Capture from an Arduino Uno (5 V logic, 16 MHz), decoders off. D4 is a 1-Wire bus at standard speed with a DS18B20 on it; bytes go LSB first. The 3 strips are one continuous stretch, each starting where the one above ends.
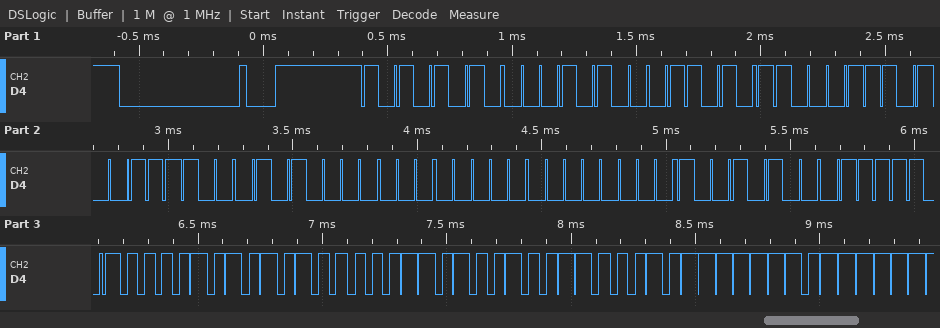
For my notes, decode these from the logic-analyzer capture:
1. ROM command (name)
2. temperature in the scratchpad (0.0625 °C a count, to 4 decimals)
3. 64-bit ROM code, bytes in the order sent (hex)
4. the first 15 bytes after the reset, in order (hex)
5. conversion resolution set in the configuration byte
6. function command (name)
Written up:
Match ROM
85.0000 °C
28 D6 B8 3C 0A 00 00 29
55 28 D6 B8 3C 0A 00 00 29 BE 50 05 4B 46 7F
12 bits
Read Scratchpad
